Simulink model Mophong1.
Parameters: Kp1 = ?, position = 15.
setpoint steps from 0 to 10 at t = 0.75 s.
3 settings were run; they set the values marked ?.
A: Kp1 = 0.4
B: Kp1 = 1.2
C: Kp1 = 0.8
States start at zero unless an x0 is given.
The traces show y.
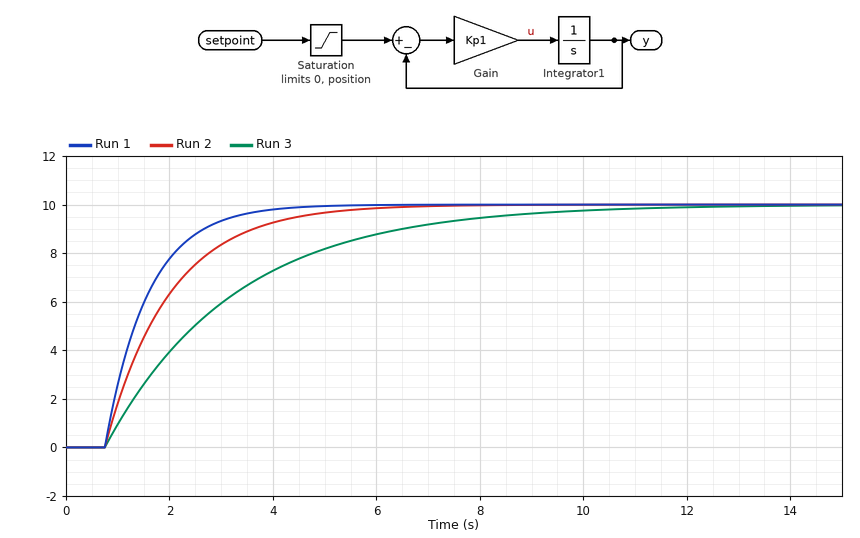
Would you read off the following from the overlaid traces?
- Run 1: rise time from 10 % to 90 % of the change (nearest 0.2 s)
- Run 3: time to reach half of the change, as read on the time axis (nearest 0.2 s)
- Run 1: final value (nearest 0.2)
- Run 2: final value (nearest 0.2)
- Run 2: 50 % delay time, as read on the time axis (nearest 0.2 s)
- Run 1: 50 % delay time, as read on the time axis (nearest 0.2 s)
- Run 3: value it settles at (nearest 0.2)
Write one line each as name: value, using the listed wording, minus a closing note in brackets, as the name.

Run 1: rise time from 10 % to 90 % of the change: 1.8 s
Run 3: time to reach half of the change, as read on the time axis: 2.4 s
Run 1: final value: 10.0
Run 2: final value: 10.0
Run 2: 50 % delay time, as read on the time axis: 1.6 s
Run 1: 50 % delay time, as read on the time axis: 1.4 s
Run 3: value it settles at: 10.0
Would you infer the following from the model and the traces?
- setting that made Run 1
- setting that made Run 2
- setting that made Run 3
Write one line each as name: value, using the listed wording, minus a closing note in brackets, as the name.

setting that made Run 1: B
setting that made Run 2: C
setting that made Run 3: A
